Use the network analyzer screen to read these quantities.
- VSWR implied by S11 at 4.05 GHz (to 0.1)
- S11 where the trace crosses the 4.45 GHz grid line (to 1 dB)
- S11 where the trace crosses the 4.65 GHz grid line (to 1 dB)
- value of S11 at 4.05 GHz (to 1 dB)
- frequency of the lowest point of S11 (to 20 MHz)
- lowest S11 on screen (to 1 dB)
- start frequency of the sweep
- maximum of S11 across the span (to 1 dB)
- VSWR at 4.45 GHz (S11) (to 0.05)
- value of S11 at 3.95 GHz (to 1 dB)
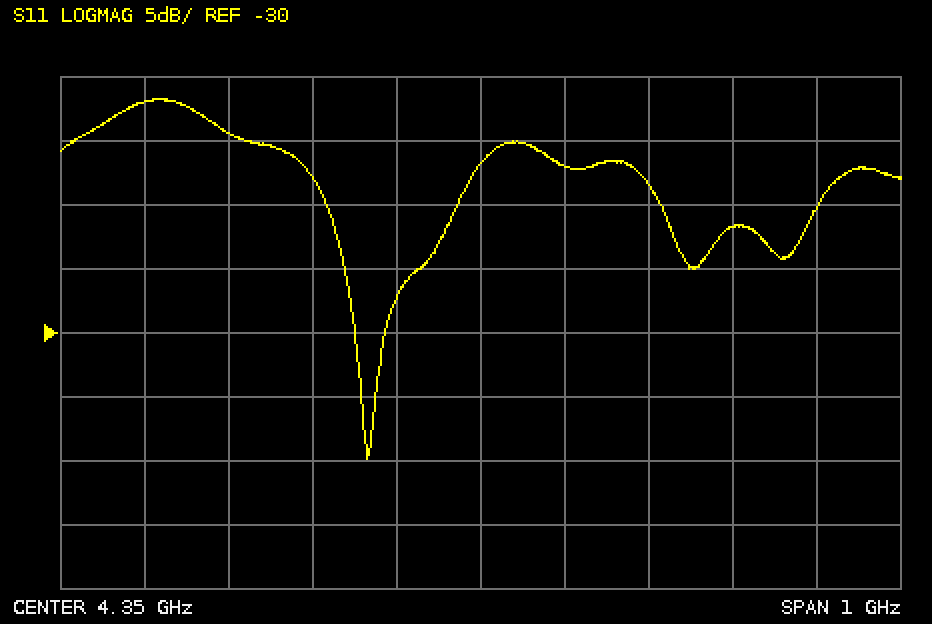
1.5
-17 dB
-22 dB
-14 dB
4.22 GHz
-40 dB
3.85 GHz
-12 dB
1.35
-12 dB
